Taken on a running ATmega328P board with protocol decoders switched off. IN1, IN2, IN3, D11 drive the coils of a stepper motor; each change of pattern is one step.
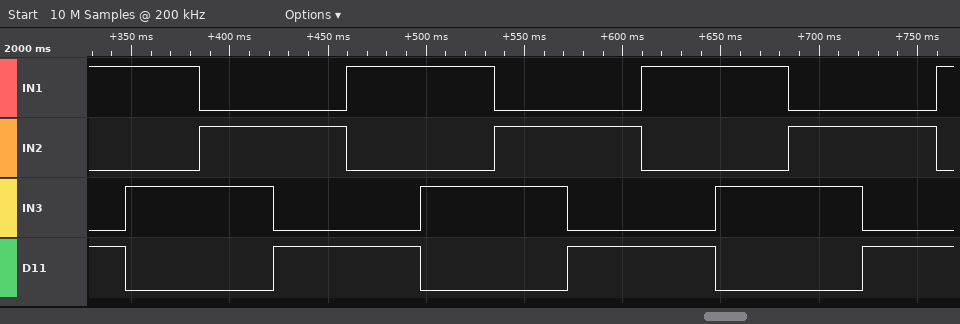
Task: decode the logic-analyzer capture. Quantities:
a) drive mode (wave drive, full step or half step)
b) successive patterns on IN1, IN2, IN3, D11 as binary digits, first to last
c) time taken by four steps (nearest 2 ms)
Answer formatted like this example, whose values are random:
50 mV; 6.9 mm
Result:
full step; 1001 1010 0110 0101 1001 1010 0110 0101 1001 1010 0110 0101 1001; 150 ms
